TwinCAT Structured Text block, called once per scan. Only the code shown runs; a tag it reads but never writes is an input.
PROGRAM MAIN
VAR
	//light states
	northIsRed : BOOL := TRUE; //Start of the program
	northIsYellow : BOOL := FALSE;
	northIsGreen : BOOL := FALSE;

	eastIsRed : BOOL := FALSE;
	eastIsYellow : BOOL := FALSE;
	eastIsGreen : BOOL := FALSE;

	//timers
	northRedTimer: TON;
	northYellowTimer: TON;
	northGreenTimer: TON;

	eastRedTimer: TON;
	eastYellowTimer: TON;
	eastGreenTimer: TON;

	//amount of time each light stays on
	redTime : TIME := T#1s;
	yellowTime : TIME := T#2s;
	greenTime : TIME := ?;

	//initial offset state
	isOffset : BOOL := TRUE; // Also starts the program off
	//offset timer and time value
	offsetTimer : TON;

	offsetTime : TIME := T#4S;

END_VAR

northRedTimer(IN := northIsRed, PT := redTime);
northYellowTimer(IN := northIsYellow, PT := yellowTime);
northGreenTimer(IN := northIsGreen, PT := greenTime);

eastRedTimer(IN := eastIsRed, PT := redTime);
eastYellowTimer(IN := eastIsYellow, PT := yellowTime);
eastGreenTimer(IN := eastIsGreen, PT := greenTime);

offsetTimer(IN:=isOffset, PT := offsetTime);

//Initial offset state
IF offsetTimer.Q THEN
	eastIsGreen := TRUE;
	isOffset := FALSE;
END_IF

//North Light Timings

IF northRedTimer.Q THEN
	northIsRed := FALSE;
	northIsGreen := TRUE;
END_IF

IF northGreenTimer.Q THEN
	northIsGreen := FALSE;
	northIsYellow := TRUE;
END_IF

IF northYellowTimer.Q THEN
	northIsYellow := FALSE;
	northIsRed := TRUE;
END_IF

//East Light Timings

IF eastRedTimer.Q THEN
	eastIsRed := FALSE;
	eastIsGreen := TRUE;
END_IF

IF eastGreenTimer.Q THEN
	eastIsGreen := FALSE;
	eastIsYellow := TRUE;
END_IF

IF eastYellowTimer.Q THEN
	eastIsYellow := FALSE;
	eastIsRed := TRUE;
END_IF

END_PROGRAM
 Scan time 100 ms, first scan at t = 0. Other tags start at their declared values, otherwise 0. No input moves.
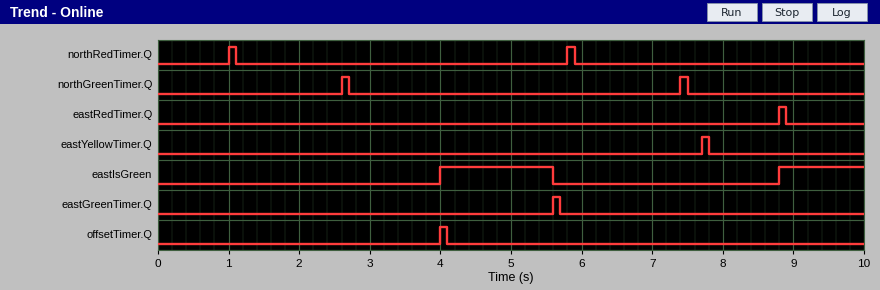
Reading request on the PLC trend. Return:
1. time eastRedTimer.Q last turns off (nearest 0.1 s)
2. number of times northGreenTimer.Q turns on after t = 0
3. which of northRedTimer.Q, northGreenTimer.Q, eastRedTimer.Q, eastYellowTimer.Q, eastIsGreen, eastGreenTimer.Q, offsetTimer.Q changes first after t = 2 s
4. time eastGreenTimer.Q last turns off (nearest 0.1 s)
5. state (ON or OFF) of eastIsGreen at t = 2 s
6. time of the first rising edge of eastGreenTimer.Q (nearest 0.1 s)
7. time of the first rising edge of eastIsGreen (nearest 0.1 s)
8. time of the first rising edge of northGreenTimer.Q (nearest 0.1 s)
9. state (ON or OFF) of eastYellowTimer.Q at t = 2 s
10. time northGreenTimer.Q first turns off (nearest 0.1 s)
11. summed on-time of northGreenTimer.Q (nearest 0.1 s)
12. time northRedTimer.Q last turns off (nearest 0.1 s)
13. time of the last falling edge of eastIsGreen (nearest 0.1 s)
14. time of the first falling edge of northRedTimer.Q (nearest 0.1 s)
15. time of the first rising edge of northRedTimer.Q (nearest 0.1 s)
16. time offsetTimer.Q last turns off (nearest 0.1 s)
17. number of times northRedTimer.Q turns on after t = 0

8.9 s
2
northGreenTimer.Q
5.7 s
OFF
5.6 s
4.0 s
2.6 s
OFF
2.7 s
0.2 s
5.9 s
5.6 s
1.1 s
1.0 s
4.1 s
2
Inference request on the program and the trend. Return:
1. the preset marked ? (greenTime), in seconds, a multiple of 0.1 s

1.5 s
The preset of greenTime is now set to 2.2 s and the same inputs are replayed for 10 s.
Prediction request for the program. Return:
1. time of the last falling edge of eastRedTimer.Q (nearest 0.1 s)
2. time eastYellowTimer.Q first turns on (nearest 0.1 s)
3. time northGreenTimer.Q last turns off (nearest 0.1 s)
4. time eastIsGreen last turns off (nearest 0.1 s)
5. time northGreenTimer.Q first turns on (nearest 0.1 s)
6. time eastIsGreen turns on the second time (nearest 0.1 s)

9.6 s
8.4 s
8.9 s
6.3 s
3.3 s
9.5 s
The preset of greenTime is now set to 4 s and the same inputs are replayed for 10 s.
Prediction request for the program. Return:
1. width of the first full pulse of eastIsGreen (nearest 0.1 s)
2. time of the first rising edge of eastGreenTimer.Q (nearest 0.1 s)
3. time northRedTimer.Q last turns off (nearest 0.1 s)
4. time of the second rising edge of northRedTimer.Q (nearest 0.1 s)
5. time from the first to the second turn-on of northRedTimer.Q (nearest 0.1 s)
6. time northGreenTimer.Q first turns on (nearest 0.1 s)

4.1 s
8.1 s
8.4 s
8.3 s
7.3 s
5.1 s
